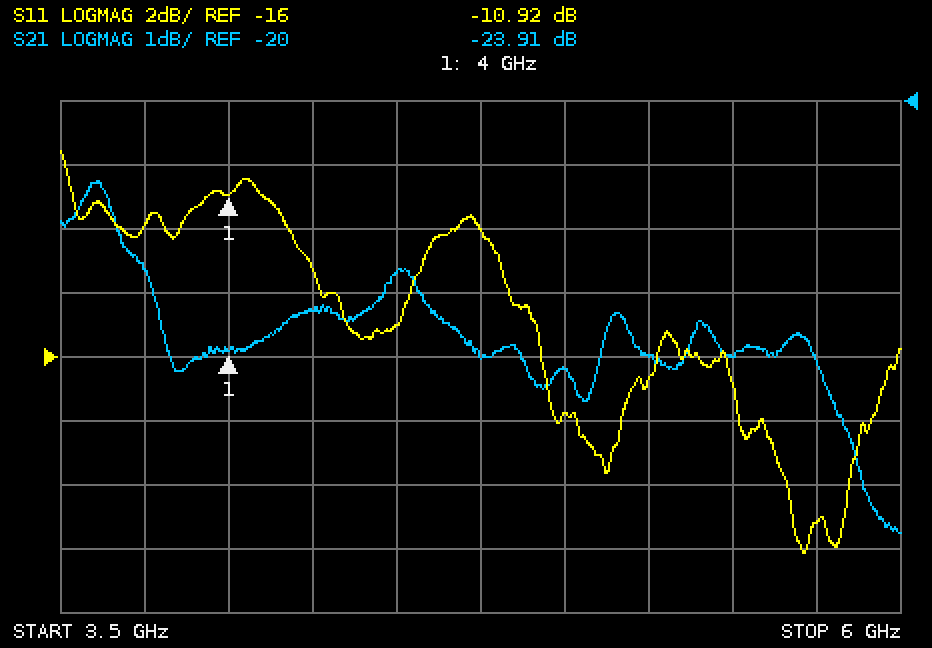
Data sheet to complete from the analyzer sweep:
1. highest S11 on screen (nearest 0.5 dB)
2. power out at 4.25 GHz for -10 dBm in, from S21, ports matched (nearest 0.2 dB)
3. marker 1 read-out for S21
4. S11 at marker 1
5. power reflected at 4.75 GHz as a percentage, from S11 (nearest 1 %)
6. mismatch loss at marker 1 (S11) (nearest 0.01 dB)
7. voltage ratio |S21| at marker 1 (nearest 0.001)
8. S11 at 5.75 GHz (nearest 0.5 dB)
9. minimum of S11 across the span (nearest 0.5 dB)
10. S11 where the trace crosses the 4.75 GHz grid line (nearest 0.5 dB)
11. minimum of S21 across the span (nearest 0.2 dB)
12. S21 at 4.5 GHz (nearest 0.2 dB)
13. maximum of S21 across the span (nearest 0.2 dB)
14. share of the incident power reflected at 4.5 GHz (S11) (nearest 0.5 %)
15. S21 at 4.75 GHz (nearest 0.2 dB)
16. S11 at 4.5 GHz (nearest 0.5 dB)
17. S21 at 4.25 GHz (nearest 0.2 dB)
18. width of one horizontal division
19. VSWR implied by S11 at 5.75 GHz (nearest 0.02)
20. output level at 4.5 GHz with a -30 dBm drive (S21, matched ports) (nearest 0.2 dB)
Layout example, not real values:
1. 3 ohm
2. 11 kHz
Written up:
1. -9.5 dB
2. -33.2 dBm
3. -23.91 dB
4. -10.92 dB
5. 6 %
6. 0.37 dB
7. 0.064
8. -21.0 dB
9. -22.0 dB
10. -12.0 dB
11. -26.8 dB
12. -22.6 dB
13. -21.2 dB
14. 3.0 %
15. -24.0 dB
16. -15.0 dB
17. -23.2 dB
18. 250 MHz
19. 1.20
20. -52.6 dBm
